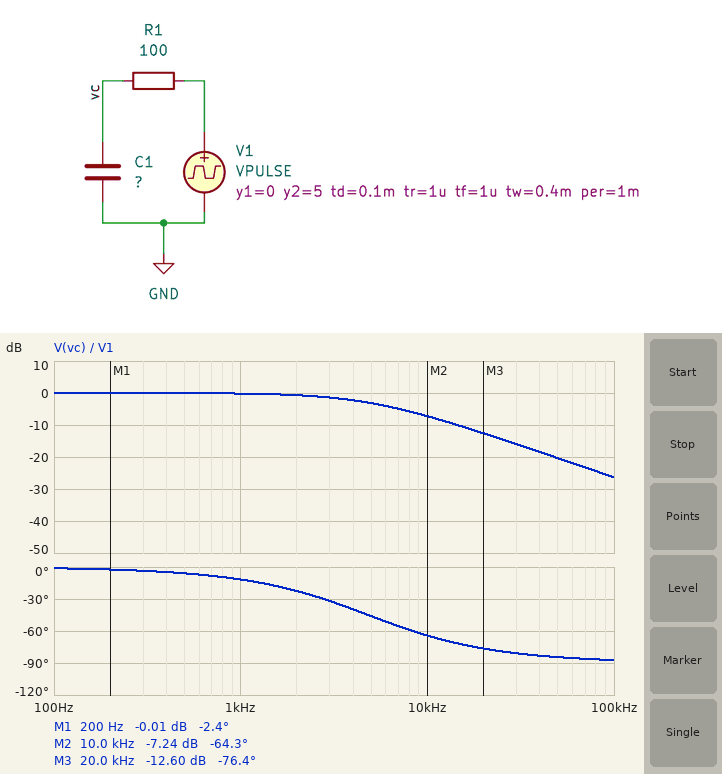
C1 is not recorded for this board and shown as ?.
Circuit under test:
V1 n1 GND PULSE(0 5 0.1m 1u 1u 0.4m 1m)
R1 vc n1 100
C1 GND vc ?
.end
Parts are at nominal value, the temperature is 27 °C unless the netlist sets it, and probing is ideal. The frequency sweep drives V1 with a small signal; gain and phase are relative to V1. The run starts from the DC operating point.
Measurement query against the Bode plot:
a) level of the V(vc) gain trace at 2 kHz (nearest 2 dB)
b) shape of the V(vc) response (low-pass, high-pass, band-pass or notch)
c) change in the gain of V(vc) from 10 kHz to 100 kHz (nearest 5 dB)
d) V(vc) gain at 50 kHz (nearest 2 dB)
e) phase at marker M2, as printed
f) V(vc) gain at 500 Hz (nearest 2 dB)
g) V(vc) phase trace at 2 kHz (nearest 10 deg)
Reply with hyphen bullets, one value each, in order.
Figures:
- 0 dB
- low-pass
- -20 dB
- -20 dB
- -64.3 deg
- 0 dB
- -20 deg
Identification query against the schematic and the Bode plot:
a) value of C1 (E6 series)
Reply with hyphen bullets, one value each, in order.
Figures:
- 330 nF
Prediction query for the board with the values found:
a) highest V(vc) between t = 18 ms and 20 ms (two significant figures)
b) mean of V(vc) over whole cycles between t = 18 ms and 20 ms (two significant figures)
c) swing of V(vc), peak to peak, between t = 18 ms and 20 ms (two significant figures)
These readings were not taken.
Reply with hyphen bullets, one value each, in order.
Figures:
- 5.0 V
- 2.0 V
- 5.0 V
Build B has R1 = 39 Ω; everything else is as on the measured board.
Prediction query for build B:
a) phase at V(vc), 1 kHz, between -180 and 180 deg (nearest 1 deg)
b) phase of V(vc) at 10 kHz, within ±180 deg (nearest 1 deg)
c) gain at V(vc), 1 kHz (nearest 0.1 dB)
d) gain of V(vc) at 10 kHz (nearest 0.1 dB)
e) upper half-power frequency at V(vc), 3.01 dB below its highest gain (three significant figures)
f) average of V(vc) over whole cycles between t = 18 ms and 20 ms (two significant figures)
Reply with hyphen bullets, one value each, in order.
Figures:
- -5 deg
- -39 deg
- 0 dB
- -2.2 dB
- 12.4 kHz
- 2.0 V
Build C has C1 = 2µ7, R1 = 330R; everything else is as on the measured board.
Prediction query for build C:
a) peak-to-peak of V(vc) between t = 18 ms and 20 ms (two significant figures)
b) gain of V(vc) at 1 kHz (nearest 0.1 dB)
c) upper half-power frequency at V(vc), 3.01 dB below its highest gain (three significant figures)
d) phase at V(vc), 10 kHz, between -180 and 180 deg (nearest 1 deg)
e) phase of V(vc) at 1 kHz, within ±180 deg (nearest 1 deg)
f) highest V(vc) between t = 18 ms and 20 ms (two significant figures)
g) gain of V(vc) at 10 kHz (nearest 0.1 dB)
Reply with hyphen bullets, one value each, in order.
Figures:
- 1.3 V
- -15.1 dB
- 179 Hz
- -89 deg
- -80 deg
- 2.7 V
- -35.0 dB
